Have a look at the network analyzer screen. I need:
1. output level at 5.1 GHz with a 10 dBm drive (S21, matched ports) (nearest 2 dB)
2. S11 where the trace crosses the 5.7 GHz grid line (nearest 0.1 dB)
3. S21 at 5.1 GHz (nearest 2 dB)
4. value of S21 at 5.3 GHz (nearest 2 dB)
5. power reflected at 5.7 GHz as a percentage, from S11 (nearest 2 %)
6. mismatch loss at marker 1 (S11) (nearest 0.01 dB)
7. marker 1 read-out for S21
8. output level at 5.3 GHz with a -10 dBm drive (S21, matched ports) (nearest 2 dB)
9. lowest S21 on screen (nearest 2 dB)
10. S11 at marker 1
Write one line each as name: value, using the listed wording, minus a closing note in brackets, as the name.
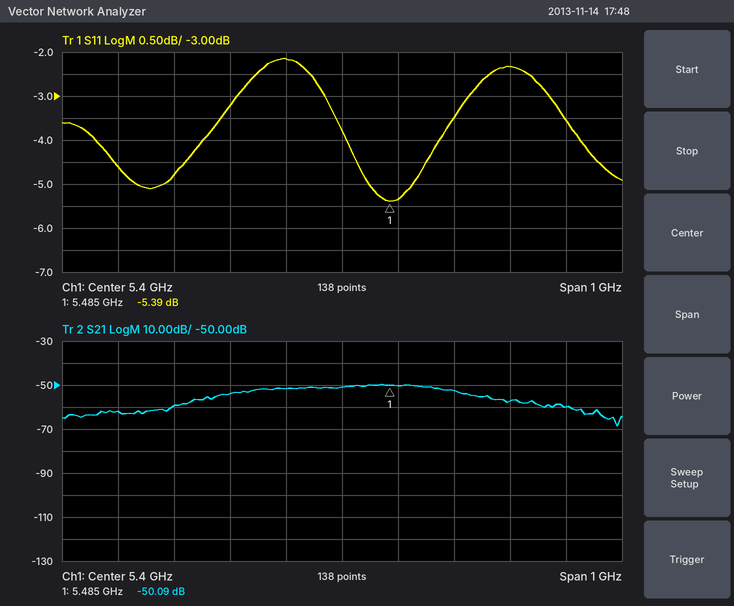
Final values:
output level at 5.1 GHz with a 10 dBm drive (S21, matched ports): -50 dBm
S11 where the trace crosses the 5.7 GHz grid line: -2.3 dB
S21 at 5.1 GHz: -60 dB
value of S21 at 5.3 GHz: -52 dB
power reflected at 5.7 GHz as a percentage, from S11: 58 %
mismatch loss at marker 1 (S11): 1.48 dB
marker 1 read-out for S21: -50.09 dB
output level at 5.3 GHz with a -10 dBm drive (S21, matched ports): -62 dBm
lowest S21 on screen: -68 dB
S11 at marker 1: -5.39 dB
